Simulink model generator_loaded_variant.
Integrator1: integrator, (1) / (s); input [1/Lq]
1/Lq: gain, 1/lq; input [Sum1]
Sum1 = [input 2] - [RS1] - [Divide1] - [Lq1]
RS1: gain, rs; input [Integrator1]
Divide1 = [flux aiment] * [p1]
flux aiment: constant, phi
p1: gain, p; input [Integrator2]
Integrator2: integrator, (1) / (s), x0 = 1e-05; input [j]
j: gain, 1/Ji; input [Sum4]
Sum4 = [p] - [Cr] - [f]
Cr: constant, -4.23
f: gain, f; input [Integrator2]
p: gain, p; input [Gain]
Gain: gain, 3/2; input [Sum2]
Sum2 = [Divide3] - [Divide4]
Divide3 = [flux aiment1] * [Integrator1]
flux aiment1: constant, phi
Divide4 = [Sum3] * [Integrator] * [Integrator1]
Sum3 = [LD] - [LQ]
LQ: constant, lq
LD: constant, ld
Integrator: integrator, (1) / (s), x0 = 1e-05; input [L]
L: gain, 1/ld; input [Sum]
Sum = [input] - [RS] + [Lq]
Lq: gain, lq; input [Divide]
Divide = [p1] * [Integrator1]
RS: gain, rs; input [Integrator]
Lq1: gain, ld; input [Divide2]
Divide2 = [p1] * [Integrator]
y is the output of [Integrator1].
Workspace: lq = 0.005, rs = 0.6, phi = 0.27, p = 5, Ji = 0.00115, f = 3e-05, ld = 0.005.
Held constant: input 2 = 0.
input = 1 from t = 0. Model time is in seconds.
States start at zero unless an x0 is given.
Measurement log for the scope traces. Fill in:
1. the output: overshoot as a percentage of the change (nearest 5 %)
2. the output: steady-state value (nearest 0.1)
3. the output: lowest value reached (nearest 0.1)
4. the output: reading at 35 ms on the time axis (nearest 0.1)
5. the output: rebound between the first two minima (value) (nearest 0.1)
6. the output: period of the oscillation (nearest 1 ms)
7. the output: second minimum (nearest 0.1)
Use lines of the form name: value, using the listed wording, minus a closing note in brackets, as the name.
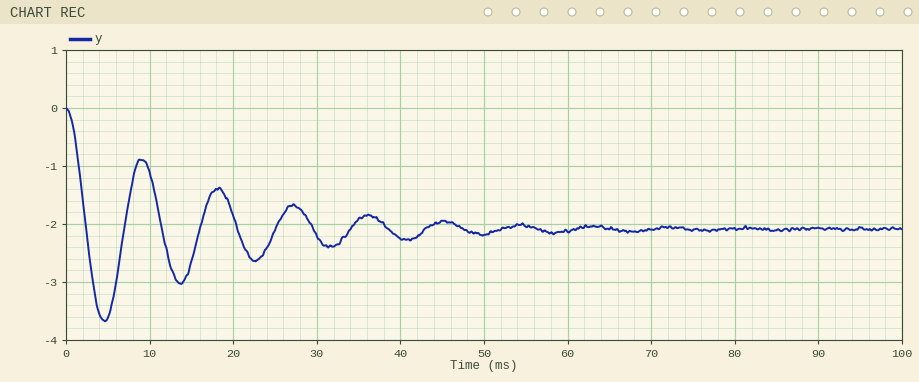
the output: overshoot as a percentage of the change: 75 %
the output: steady-state value: -2.1
the output: lowest value reached: -3.7
the output: reading at 35 ms on the time axis: -1.9
the output: rebound between the first two minima (value): -0.9
the output: period of the oscillation: 9 ms
the output: second minimum: -3.0
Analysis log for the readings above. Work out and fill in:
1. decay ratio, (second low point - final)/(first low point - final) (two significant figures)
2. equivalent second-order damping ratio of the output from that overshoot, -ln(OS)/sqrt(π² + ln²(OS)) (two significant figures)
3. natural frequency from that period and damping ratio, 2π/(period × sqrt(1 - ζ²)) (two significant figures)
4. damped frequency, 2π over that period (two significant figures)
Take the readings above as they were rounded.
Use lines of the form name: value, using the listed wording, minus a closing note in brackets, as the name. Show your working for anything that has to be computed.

decay ratio, (second low point - final)/(first low point - final): (-3 - (-2.1)) / (-3.7 - (-2.1)) = 0.56
equivalent second-order damping ratio of the output from that overshoot, -ln(OS)/sqrt(π² + ln²(OS)): ln(0.75) = -0.288; 0.288 / sqrt(9.870 + 0.083) = 0.091
natural frequency from that period and damping ratio, 2π/(period × sqrt(1 - ζ²)): 2π / (9 × sqrt(1 - 0.091²)) = 0.70 rad/ms
damped frequency, 2π over that period: 2π / 9 = 0.70 rad/ms
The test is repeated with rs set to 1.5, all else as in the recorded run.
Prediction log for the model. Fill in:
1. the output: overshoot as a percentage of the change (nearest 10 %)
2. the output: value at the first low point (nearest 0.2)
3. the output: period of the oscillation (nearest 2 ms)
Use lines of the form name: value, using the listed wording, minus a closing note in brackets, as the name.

the output: overshoot as a percentage of the change: 50 %
the output: value at the first low point: -3.2
the output: period of the oscillation: 10 ms
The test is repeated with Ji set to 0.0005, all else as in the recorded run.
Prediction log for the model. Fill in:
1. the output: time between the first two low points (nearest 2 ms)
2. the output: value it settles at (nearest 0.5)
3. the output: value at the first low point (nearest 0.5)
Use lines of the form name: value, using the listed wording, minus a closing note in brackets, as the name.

the output: time between the first two low points: 6 ms
the output: value it settles at: -2.0
the output: value at the first low point: -4.0
